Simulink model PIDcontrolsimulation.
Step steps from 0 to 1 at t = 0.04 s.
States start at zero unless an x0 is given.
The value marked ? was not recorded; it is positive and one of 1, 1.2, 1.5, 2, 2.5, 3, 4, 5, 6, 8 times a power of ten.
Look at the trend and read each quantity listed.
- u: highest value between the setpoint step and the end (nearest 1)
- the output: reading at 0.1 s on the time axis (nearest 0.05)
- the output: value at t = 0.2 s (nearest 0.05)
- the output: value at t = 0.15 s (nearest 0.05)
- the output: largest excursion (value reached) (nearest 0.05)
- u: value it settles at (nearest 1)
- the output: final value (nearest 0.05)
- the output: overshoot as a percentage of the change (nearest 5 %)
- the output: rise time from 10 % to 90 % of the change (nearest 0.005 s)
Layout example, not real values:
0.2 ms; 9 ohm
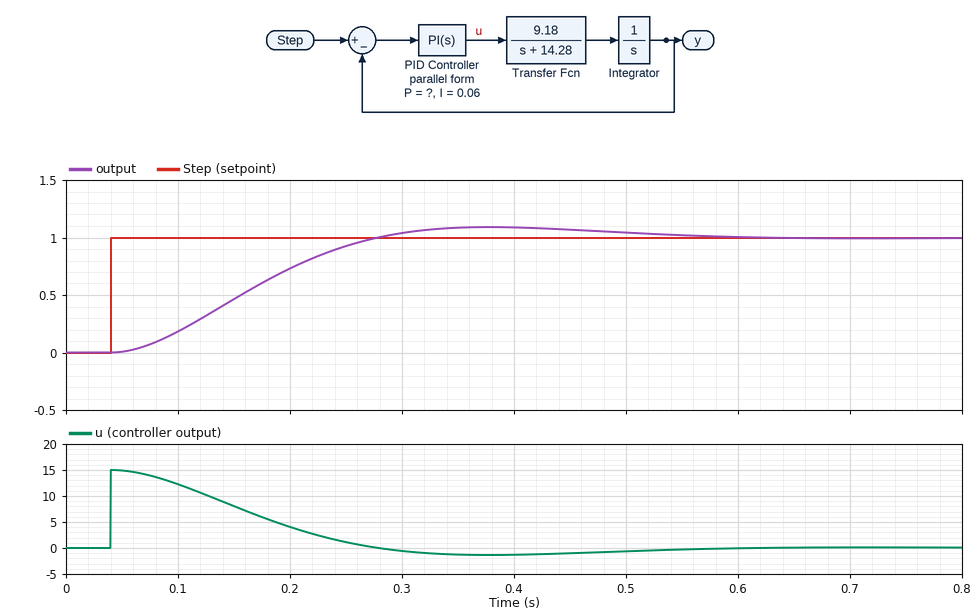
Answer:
15; 0.20; 0.75; 0.45; 1.10; 0; 1.00; 10 %; 0.160 s
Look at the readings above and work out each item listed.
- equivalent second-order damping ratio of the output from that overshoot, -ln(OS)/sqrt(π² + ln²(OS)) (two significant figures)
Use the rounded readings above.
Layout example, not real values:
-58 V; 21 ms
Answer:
0.59
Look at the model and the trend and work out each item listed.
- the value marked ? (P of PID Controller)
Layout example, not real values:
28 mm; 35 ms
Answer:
15
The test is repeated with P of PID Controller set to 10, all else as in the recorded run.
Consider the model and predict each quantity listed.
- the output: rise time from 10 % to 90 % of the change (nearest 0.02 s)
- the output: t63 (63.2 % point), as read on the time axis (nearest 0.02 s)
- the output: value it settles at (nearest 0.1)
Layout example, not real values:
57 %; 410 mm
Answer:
0.24 s; 0.22 s; 1.0
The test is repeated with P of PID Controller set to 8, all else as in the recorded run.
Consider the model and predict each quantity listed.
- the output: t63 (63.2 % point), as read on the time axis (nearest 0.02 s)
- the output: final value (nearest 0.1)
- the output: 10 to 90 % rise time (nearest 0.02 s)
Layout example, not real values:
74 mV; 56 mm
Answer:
0.26 s; 1.0; 0.30 s
